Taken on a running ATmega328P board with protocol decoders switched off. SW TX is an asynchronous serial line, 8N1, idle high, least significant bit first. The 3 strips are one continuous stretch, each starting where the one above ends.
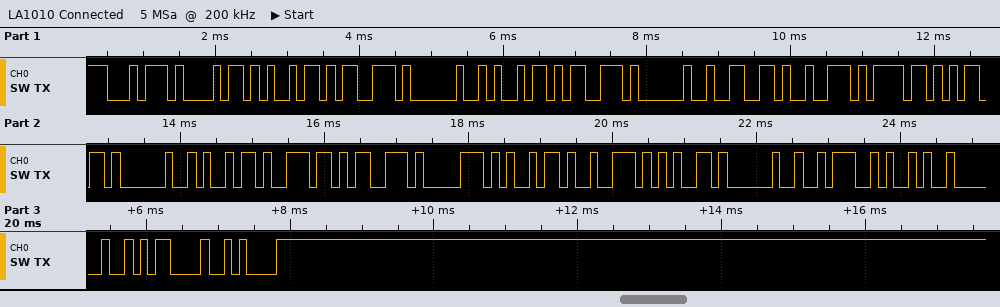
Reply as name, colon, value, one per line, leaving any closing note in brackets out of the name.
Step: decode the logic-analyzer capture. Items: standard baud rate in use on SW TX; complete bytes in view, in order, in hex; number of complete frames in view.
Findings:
standard baud rate in use on SW TX: 9600 baud
complete bytes in view, in order, in hex: 74 68 69 73 20 69 73 20 66 72 6F 6D 20 69 6E 73 70 69 72 65 20 3A 29 20 0D 0A
number of complete frames in view: 26
